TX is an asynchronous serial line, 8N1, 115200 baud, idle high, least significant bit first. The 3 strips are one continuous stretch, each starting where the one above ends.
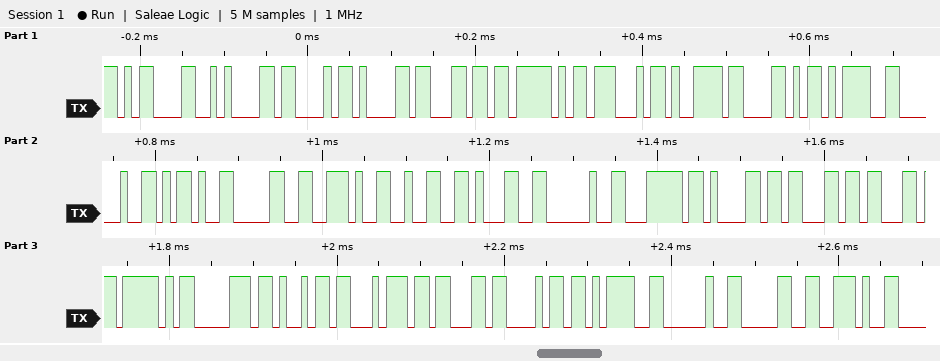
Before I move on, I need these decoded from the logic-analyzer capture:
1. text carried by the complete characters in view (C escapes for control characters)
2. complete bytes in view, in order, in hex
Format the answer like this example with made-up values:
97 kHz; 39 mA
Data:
"\r\nCal_GyX= -0.21 |acc_pitch= 0."; 0D 0A 43 61 6C 5F 47 79 58 3D 20 2D 30 2E 32 31 20 7C 61 63 63 5F 70 69 74 63 68 3D 20 30 2E
